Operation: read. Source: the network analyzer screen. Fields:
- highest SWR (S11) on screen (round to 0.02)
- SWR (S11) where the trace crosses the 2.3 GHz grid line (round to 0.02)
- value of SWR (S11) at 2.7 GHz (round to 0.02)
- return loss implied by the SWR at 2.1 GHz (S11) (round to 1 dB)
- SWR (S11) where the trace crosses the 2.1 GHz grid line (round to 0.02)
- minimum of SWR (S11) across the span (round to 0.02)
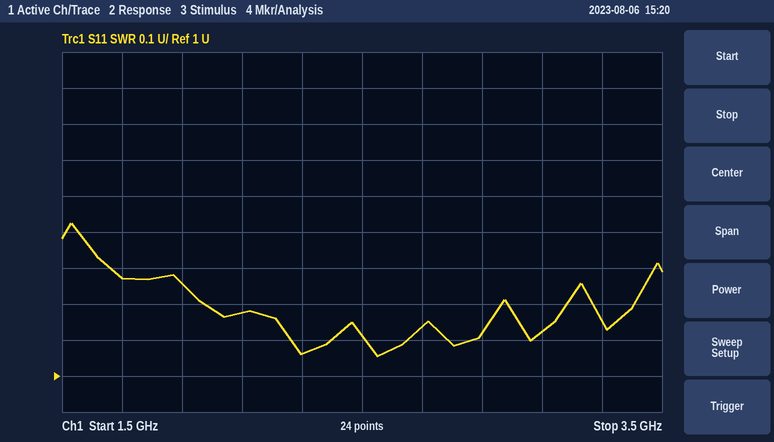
1.42
1.06
1.14
22 dB
1.18
1.06
